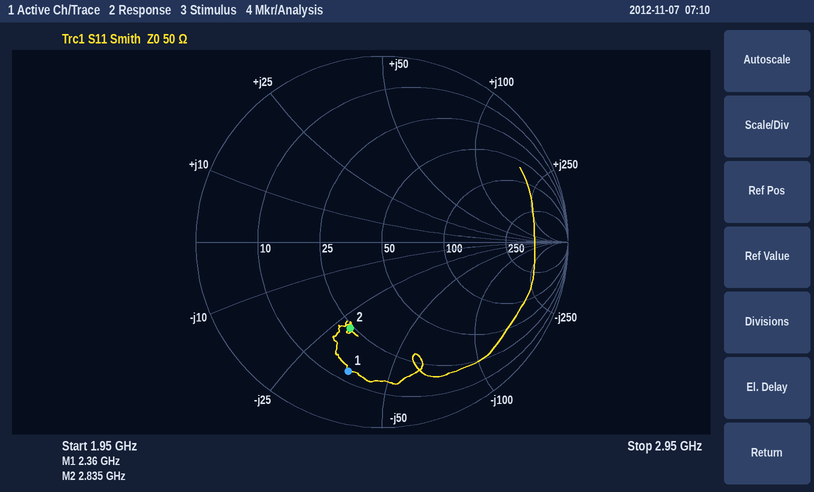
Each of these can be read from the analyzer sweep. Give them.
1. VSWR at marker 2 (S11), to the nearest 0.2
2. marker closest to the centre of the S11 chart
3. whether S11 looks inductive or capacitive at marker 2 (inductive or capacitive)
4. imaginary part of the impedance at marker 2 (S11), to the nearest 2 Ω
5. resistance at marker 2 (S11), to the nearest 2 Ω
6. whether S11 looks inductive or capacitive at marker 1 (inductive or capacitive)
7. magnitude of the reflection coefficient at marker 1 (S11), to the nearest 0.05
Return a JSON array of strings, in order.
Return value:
["3.0", "marker 2", "capacitive", "-30 Ω", "24 Ω", "capacitive", "0.70"]
